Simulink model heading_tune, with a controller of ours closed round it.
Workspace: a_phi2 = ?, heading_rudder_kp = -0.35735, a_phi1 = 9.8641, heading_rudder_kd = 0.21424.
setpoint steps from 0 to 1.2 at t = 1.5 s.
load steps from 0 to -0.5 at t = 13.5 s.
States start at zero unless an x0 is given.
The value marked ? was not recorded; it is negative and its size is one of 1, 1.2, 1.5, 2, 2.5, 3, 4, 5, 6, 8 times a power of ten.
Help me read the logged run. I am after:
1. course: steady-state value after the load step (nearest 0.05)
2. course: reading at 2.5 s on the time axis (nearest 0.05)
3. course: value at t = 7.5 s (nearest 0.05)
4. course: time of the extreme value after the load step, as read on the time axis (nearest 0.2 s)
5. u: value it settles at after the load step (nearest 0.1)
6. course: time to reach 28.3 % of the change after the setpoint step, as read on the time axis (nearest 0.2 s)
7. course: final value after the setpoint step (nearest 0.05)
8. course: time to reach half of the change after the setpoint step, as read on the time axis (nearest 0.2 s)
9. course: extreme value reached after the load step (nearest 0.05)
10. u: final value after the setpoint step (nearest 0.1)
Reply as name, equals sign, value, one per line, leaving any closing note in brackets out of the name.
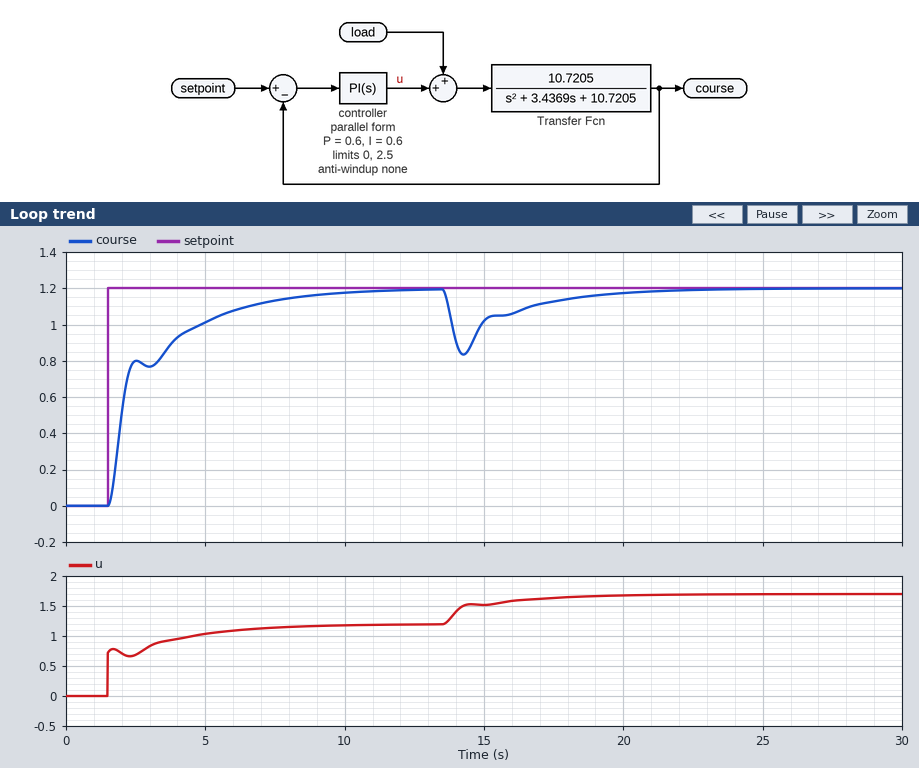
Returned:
course: steady-state value after the load step = 1.20
course: reading at 2.5 s on the time axis = 0.80
course: value at t = 7.5 s = 1.15
course: time of the extreme value after the load step, as read on the time axis = 14.2 s
u: value it settles at after the load step = 1.7
course: time to reach 28.3 % of the change after the setpoint step, as read on the time axis = 1.8 s
course: final value after the setpoint step = 1.20
course: time to reach half of the change after the setpoint step, as read on the time axis = 2.0 s
course: extreme value reached after the load step = 0.85
u: final value after the setpoint step = 1.2
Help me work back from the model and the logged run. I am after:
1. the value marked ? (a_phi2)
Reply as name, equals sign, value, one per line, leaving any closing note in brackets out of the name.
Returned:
the value marked ? = -30
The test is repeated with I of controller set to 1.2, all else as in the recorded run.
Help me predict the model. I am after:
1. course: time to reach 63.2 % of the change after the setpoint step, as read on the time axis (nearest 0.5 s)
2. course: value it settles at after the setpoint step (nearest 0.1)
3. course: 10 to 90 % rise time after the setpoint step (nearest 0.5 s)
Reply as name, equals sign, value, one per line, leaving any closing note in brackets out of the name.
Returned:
course: time to reach 63.2 % of the change after the setpoint step, as read on the time axis = 2.0 s
course: value it settles at after the setpoint step = 1.2
course: 10 to 90 % rise time after the setpoint step = 2.0 s
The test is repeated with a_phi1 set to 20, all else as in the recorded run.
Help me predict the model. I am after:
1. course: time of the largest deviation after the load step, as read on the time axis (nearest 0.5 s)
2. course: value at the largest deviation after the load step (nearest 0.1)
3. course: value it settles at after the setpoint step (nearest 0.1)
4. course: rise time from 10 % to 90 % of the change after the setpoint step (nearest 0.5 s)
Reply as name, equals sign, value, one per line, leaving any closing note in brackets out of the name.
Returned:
course: time of the largest deviation after the load step, as read on the time axis = 15.0 s
course: value at the largest deviation after the load step = 1.0
course: value it settles at after the setpoint step = 1.2
course: rise time from 10 % to 90 % of the change after the setpoint step = 3.5 s
